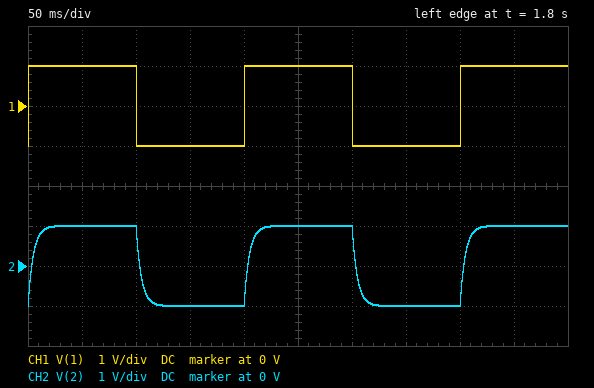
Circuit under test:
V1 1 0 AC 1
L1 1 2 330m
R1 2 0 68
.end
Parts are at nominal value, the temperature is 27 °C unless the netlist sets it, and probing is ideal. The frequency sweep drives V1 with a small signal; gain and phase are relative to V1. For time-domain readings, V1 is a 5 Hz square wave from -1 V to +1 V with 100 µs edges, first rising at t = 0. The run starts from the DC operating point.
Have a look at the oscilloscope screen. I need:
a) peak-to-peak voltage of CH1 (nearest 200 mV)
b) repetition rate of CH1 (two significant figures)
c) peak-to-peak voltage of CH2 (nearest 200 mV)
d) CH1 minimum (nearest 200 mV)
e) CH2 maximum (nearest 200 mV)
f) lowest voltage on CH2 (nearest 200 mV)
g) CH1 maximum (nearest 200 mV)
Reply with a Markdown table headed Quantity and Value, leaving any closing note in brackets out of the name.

| Quantity | Value |
|---|---|
| peak-to-peak voltage of CH1 | 2.0 V |
| repetition rate of CH1 | 5.0 Hz |
| peak-to-peak voltage of CH2 | 2.0 V |
| CH1 minimum | -1.0 V |
| CH2 maximum | 1.0 V |
| lowest voltage on CH2 | -1.0 V |
| CH1 maximum | 1.0 V |
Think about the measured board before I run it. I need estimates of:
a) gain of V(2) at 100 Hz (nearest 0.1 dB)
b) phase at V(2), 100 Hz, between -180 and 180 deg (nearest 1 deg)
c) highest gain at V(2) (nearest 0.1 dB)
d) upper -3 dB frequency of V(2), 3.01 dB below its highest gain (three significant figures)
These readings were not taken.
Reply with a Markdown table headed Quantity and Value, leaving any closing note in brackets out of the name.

| Quantity | Value |
|---|---|
| gain of V(2) at 100 Hz | -10.1 dB |
| phase at V(2), 100 Hz, between -180 and 180 deg | -72 deg |
| highest gain at V(2) | 0 dB |
| upper -3 dB frequency of V(2), 3.01 dB below its highest gain | 32.8 Hz |
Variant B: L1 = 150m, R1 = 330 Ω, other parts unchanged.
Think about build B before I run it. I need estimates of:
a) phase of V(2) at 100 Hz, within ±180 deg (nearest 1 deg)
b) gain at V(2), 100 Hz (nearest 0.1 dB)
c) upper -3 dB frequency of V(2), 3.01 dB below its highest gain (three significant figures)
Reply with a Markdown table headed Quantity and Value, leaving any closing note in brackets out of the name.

| Quantity | Value |
|---|---|
| phase of V(2) at 100 Hz, within ±180 deg | -16 deg |
| gain at V(2), 100 Hz | -0.3 dB |
| upper -3 dB frequency of V(2), 3.01 dB below its highest gain | 350 Hz |
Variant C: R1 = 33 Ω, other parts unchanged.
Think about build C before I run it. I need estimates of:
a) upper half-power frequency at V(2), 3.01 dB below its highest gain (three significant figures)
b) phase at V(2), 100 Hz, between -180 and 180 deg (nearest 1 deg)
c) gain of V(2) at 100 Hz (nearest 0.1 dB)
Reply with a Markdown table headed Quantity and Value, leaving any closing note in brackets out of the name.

| Quantity | Value |
|---|---|
| upper half-power frequency at V(2), 3.01 dB below its highest gain | 15.9 Hz |
| phase at V(2), 100 Hz, between -180 and 180 deg | -81 deg |
| gain of V(2) at 100 Hz | -16.1 dB |
